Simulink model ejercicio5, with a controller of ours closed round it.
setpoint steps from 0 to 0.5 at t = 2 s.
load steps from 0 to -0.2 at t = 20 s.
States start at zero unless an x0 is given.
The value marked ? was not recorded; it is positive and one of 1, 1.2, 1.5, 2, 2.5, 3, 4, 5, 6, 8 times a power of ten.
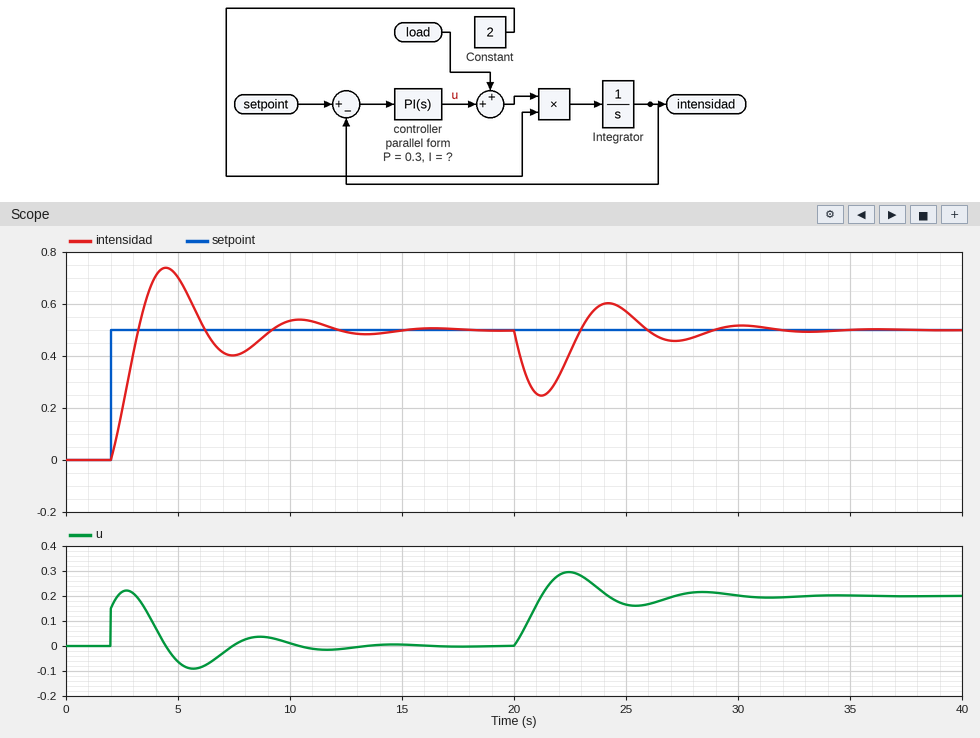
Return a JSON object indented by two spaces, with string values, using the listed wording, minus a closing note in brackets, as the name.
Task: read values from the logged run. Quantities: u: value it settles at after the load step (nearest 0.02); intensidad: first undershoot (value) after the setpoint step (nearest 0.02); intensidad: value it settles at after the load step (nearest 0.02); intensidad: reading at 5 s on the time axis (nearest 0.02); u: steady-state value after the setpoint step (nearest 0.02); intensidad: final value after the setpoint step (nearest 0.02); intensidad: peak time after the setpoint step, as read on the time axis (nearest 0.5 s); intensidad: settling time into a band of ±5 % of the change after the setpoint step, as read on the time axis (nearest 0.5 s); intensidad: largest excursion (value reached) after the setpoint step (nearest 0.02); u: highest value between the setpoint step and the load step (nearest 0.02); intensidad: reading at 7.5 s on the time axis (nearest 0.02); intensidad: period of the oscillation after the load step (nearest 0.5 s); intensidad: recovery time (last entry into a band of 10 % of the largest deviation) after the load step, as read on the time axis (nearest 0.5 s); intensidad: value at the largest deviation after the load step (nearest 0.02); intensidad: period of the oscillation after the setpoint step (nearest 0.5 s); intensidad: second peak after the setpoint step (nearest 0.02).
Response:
{
  "u: value it settles at after the load step": "0.20",
  "intensidad: first undershoot (value) after the setpoint step": "0.40",
  "intensidad: value it settles at after the load step": "0.50",
  "intensidad: reading at 5 s on the time axis": "0.70",
  "u: steady-state value after the setpoint step": "0.00",
  "intensidad: final value after the setpoint step": "0.50",
  "intensidad: peak time after the setpoint step, as read on the time axis": "4.5 s",
  "intensidad: settling time into a band of ±5 % of the change after the setpoint step, as read on the time axis": "11.5 s",
  "intensidad: largest excursion (value reached) after the setpoint step": "0.74",
  "u: highest value between the setpoint step and the load step": "0.22",
  "intensidad: reading at 7.5 s on the time axis": "0.40",
  "intensidad: period of the oscillation after the load step": "6.0 s",
  "intensidad: recovery time (last entry into a band of 10 % of the largest deviation) after the load step, as read on the time axis": "28.0 s",
  "intensidad: value at the largest deviation after the load step": "0.24",
  "intensidad: period of the oscillation after the setpoint step": "6.0 s",
  "intensidad: second peak after the setpoint step": "0.54"
}
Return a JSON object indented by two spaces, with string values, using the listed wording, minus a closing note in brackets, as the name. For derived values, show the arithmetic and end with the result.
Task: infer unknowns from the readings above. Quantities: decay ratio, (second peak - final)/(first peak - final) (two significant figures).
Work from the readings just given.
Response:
{
  "decay ratio, (second peak - final)/(first peak - final)": "(0.54 - 0.5) / (0.74 - 0.5) = 0.17"
}
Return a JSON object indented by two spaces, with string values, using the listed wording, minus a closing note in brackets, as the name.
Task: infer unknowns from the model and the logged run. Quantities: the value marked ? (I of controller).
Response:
{
  "the value marked ?": "0.6"
}
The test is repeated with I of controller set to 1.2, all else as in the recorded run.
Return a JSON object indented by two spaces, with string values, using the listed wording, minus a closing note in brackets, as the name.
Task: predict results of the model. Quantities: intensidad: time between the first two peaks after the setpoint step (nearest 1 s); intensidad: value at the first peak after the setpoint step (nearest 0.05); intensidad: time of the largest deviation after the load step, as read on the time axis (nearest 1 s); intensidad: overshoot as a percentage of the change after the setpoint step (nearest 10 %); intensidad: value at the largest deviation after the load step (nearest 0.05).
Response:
{
  "intensidad: time between the first two peaks after the setpoint step": "4 s",
  "intensidad: value at the first peak after the setpoint step": "0.80",
  "intensidad: time of the largest deviation after the load step, as read on the time axis": "21 s",
  "intensidad: overshoot as a percentage of the change after the setpoint step": "60 %",
  "intensidad: value at the largest deviation after the load step": "0.30"
}
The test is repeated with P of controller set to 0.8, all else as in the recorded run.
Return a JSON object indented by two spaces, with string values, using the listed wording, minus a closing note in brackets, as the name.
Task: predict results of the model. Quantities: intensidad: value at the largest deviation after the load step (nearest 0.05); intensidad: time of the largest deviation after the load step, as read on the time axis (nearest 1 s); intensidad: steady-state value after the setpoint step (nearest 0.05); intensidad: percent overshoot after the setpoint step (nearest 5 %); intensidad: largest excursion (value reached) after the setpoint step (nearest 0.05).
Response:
{
  "intensidad: value at the largest deviation after the load step": "0.35",
  "intensidad: time of the largest deviation after the load step, as read on the time axis": "21 s",
  "intensidad: steady-state value after the setpoint step": "0.50",
  "intensidad: percent overshoot after the setpoint step": "20 %",
  "intensidad: largest excursion (value reached) after the setpoint step": "0.60"
}
